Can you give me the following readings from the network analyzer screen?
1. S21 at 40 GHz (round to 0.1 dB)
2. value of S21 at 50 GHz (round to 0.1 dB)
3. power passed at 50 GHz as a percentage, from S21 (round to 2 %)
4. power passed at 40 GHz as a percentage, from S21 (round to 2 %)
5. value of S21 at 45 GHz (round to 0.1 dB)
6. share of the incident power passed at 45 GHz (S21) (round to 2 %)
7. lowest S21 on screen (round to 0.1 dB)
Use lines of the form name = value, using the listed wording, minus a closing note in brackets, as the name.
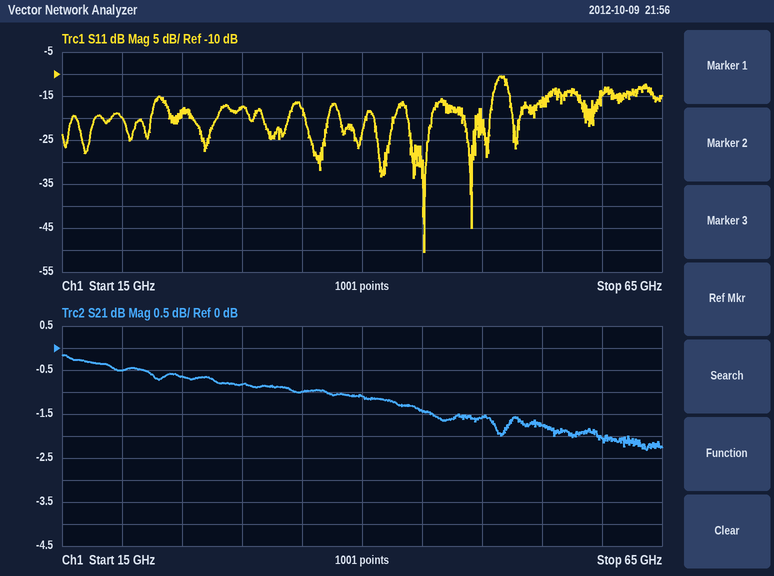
S21 at 40 GHz = -1.1 dB
value of S21 at 50 GHz = -1.6 dB
power passed at 50 GHz as a percentage, from S21 = 70 %
power passed at 40 GHz as a percentage, from S21 = 78 %
value of S21 at 45 GHz = -1.4 dB
share of the incident power passed at 45 GHz (S21) = 72 %
lowest S21 on screen = -2.3 dB
